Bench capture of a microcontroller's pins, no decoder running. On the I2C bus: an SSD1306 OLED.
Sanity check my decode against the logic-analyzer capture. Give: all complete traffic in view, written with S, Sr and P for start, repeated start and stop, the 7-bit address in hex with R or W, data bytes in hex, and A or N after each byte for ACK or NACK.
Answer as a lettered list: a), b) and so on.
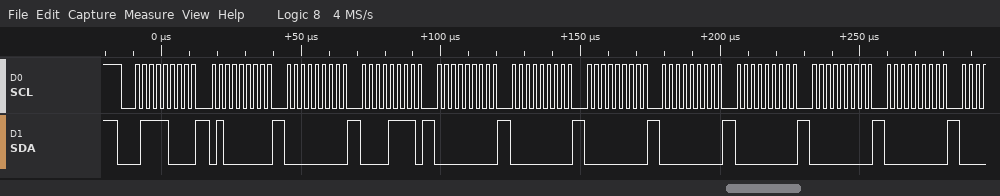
a) S 3CW A 40 A 00 A 0F A 00 A 00 A 00 A 00 A 00 A 00 A 00 A
